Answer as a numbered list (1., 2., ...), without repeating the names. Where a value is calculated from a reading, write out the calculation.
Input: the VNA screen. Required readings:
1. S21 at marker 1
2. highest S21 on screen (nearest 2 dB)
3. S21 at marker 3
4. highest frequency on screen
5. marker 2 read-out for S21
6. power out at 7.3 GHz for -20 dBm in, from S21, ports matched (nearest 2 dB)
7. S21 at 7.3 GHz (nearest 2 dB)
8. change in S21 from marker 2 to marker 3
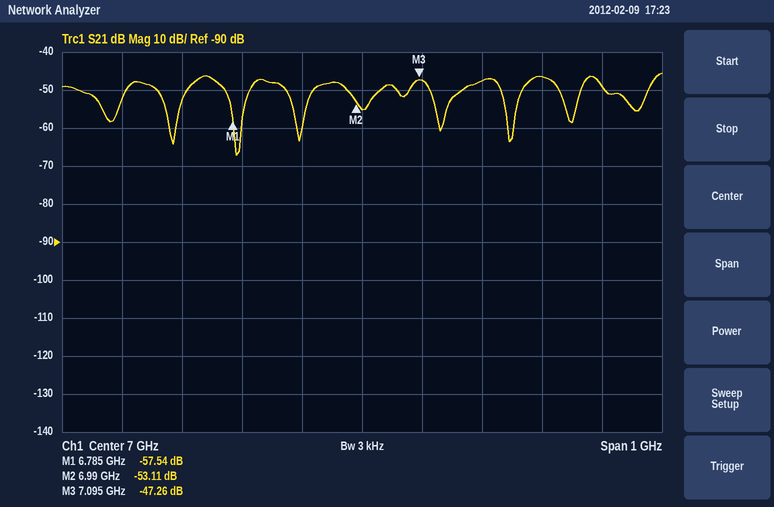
1. -57.54 dB
2. -46 dB
3. -47.26 dB
4. 7.5 GHz
5. -53.11 dB
6. -20 dBm + (-46 dB) = -66 dBm
7. -46 dB
8. -47.26 − (-53.11) = 5.85 dB
